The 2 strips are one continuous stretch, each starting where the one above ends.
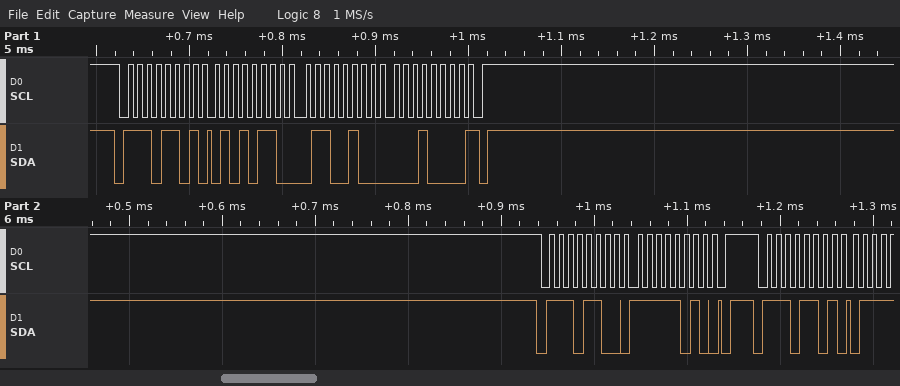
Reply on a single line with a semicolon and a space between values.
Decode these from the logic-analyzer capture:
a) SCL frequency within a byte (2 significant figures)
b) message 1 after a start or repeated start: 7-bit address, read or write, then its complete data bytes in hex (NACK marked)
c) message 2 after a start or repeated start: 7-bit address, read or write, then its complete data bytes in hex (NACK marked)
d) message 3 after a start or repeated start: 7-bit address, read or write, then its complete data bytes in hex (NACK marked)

100 kHz; 0x76 read: 56 64 10 NACK; 0x76 write: FA; 0x76 read
